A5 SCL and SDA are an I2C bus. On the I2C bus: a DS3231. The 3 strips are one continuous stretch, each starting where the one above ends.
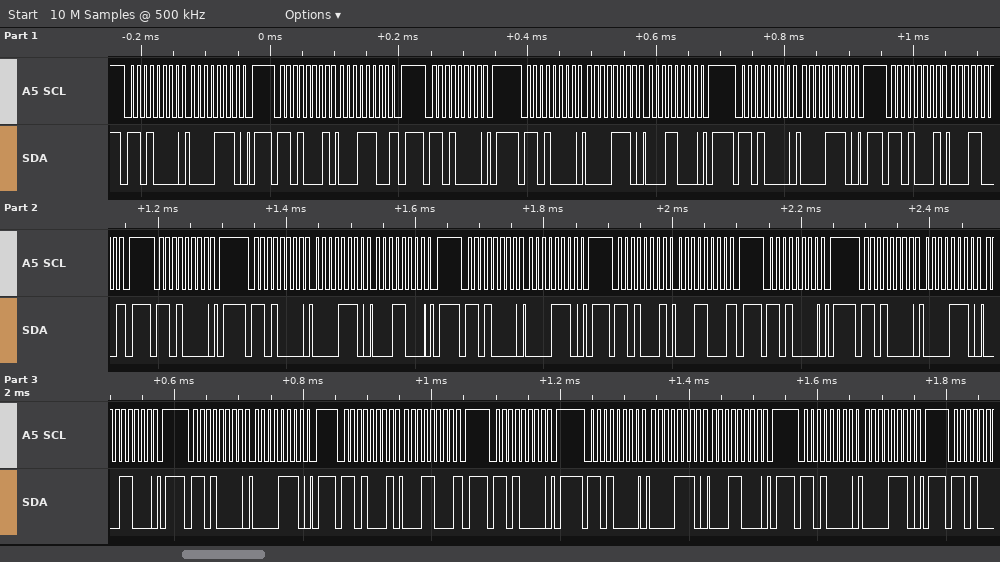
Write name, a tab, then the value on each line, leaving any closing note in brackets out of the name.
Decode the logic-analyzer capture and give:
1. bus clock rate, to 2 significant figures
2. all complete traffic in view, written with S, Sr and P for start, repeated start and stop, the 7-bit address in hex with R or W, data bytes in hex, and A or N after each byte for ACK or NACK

bus clock rate, to 2 significant figures	100 kHz
all complete traffic in view, written with S, Sr and P for start, repeated start and stop, the 7-bit address in hex with R or W, data bytes in hex, and A or N after each byte for ACK or NACK	S 68W A 0E A P S 68R A 1C N P S 68W A P S 68W A 0E A 18 A P S 68W A 0E A P S 68R A 18 N P S 68W A P S 68W A 0E A 18 A P S 68W A 0E A P S 68R A 18 N P S 68W A P S 68W A 0E A 18 A P S 68W A 0E A P S 68R A 18 N P S 68W A P S 68W A 0E A 18 A P S 68W A 0E A P
